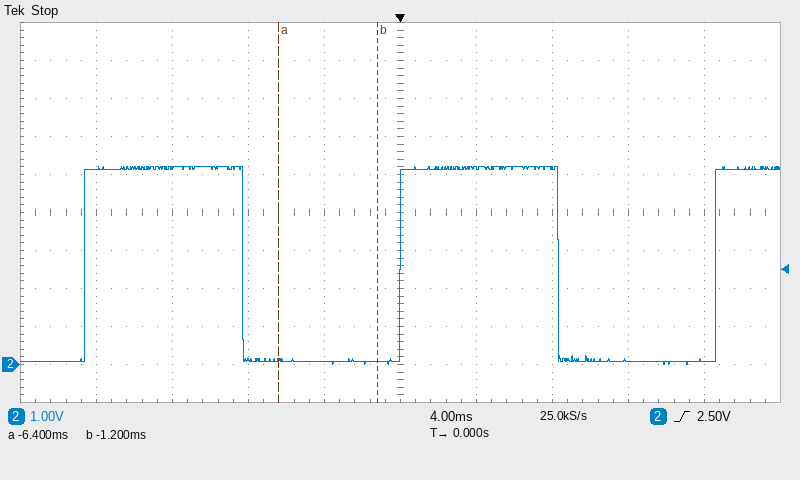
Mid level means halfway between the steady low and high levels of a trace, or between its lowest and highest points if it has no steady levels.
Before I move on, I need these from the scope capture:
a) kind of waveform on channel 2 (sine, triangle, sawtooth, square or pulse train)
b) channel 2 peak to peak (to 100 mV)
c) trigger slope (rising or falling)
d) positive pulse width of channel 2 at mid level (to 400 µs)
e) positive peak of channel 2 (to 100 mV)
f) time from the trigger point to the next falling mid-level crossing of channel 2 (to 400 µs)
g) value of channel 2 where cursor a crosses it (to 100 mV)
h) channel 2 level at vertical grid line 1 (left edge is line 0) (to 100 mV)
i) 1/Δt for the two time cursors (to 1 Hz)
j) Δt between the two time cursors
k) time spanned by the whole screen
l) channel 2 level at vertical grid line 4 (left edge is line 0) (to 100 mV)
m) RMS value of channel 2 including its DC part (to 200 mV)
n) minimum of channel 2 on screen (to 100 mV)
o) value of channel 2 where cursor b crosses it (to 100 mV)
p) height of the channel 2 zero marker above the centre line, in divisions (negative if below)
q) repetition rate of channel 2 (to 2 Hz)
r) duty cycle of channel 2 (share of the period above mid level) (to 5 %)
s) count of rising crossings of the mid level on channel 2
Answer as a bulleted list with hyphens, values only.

- square
- 5.2 V
- rising
- 8.4 ms
- 5.2 V
- 8.4 ms
- 100 mV
- 5.2 V
- 192 Hz
- 5.2 ms
- 40 ms
- 100 mV
- 3.6 V
- 0.0 V
- 100 mV
- -4.0 div
- 60 Hz
- 50 %
- 3
